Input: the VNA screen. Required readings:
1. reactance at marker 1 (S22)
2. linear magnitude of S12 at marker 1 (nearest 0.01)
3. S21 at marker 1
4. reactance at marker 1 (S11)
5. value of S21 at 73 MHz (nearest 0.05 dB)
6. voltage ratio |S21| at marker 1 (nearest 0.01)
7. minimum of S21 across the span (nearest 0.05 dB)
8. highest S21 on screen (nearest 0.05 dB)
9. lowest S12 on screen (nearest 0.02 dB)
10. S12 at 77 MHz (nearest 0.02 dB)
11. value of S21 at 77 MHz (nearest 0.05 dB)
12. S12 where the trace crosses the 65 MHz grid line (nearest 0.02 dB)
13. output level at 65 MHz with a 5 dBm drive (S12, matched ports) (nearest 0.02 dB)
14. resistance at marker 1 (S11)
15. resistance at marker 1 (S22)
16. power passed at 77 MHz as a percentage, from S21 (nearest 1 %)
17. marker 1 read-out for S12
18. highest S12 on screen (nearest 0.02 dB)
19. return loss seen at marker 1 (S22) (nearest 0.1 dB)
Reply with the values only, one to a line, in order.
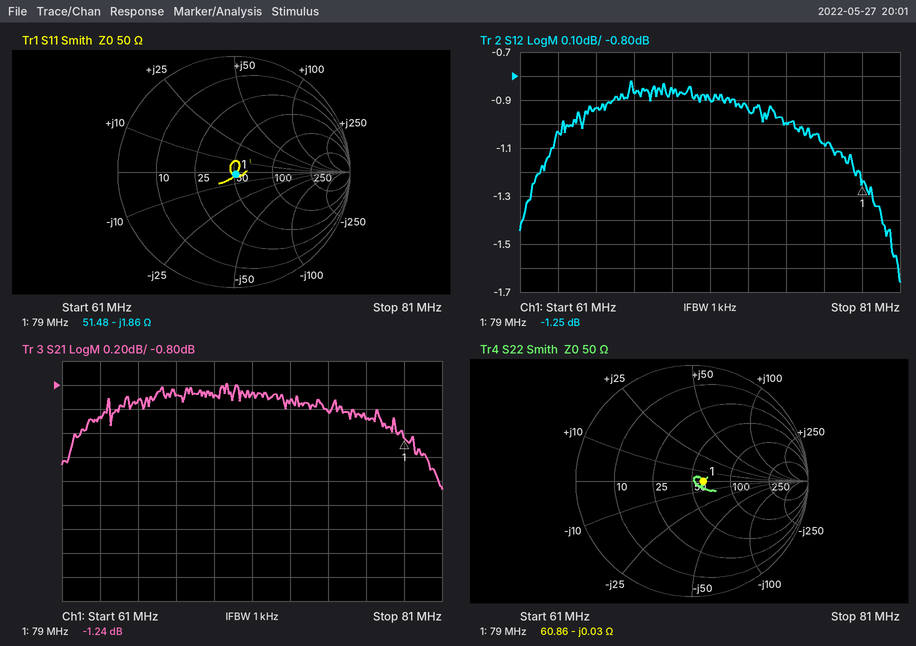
-0.03 Ω
0.87
-1.24 dB
-1.86 Ω
-0.95 dB
0.87
-1.65 dB
-0.80 dB
-1.66 dB
-1.08 dB
-1.10 dB
-0.94 dB
4.06 dBm
51.48 Ω
60.86 Ω
78 %
-1.25 dB
-0.82 dB
20.2 dB
